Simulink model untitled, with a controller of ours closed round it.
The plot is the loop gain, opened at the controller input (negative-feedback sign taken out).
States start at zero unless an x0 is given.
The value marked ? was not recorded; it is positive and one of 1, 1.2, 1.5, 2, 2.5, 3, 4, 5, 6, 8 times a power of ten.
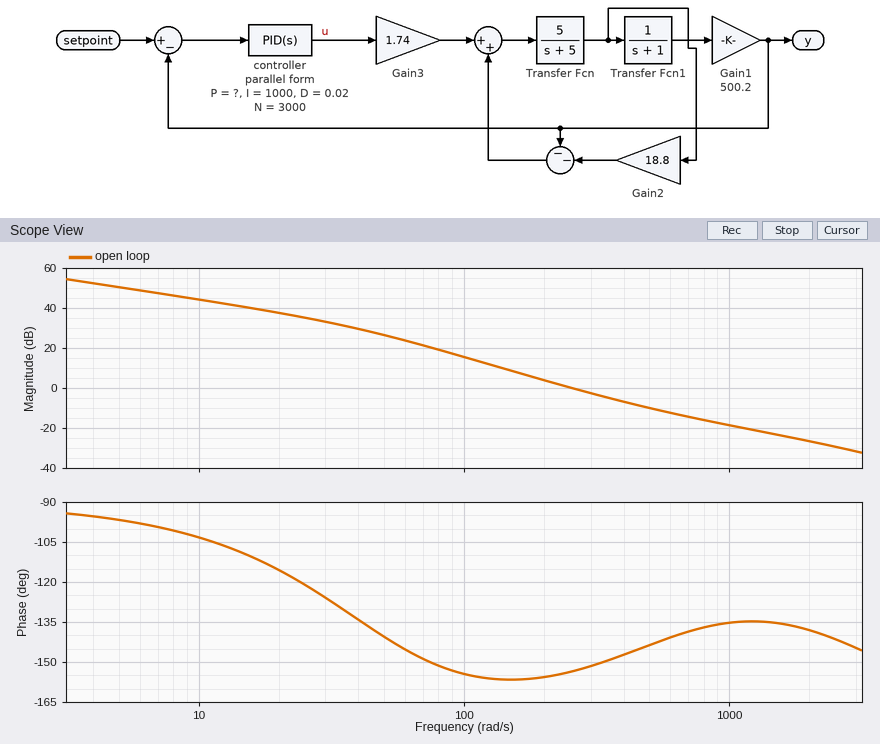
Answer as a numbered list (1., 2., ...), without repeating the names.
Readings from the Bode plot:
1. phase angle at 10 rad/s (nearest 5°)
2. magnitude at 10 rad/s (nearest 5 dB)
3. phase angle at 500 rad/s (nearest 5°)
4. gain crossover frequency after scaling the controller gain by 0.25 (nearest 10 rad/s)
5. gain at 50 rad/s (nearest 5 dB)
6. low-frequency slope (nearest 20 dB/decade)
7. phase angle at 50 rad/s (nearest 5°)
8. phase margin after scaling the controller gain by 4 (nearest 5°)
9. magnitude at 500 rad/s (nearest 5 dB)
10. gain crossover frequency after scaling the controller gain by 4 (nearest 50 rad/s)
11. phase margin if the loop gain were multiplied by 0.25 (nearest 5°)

1. -105°
2. 45 dB
3. -145°
4. 120 rad/s
5. 25 dB
6. -20 dB/decade
7. -140°
8. 40°
9. -10 dB
10. 600 rad/s
11. 25°
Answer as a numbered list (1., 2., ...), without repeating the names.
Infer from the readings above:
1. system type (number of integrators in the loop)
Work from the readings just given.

1. 1
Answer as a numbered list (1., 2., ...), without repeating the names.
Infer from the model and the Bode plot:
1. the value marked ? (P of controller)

1. 15
